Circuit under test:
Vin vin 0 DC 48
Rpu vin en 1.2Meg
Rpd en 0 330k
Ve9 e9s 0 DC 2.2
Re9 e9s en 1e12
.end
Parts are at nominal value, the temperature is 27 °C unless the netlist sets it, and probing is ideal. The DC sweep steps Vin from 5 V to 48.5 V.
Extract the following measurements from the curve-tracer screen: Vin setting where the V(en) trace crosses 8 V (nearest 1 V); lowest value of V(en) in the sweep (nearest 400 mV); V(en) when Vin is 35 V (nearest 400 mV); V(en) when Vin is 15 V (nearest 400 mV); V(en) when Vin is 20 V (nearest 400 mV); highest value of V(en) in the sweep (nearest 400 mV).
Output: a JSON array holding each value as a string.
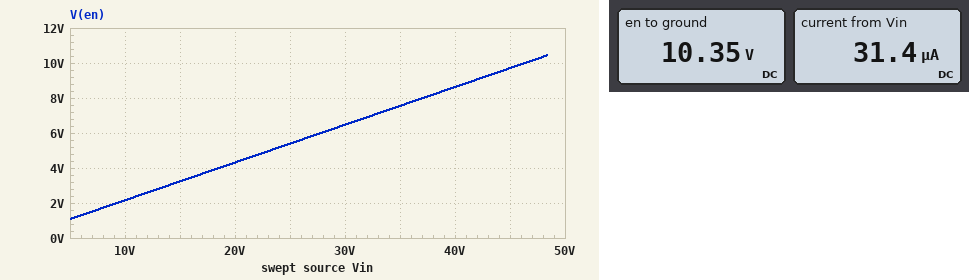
["37 V", "1.2 V", "7.6 V", "3.2 V", "4.4 V", "10.4 V"]
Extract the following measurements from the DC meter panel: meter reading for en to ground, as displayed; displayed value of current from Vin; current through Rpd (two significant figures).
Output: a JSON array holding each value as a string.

["10.35 V", "31.4 µA", "31 µA"]
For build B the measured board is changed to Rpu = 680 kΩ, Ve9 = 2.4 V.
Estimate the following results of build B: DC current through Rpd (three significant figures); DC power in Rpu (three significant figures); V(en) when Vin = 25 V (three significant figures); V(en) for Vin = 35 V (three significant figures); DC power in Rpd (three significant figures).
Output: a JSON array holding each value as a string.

["47.5 µA", "1.54 mW", "8.17 V", "11.4 V", "745 µW"]
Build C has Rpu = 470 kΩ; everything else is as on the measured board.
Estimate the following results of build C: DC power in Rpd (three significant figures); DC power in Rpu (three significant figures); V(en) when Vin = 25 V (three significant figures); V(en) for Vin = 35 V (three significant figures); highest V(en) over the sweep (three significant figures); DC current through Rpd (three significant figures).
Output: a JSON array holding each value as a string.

["1.19 mW", "1.69 mW", "10.3 V", "14.4 V", "20.0 V", "60.0 µA"]
